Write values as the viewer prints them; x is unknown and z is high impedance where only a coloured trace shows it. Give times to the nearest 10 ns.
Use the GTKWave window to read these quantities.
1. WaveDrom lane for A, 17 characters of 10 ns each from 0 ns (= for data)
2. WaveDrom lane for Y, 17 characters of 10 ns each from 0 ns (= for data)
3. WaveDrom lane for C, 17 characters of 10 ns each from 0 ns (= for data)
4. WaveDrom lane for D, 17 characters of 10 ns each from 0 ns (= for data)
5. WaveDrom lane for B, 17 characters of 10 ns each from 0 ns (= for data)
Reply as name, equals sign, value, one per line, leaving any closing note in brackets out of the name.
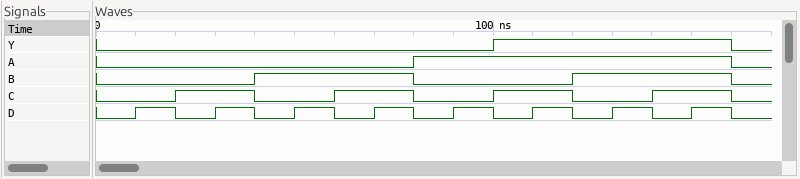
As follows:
WaveDrom lane for A, 17 characters of 10 ns each from 0 ns = {name: 'A', wave: '0.......1.......0'}
WaveDrom lane for Y, 17 characters of 10 ns each from 0 ns = {name: 'Y', wave: '0.........1.....0'}
WaveDrom lane for C, 17 characters of 10 ns each from 0 ns = {name: 'C', wave: '0.1.0.1.0.1.0.1.0'}
WaveDrom lane for D, 17 characters of 10 ns each from 0 ns = {name: 'D', wave: '01010101010101010'}
WaveDrom lane for B, 17 characters of 10 ns each from 0 ns = {name: 'B', wave: '0...1...0...1...0'}
